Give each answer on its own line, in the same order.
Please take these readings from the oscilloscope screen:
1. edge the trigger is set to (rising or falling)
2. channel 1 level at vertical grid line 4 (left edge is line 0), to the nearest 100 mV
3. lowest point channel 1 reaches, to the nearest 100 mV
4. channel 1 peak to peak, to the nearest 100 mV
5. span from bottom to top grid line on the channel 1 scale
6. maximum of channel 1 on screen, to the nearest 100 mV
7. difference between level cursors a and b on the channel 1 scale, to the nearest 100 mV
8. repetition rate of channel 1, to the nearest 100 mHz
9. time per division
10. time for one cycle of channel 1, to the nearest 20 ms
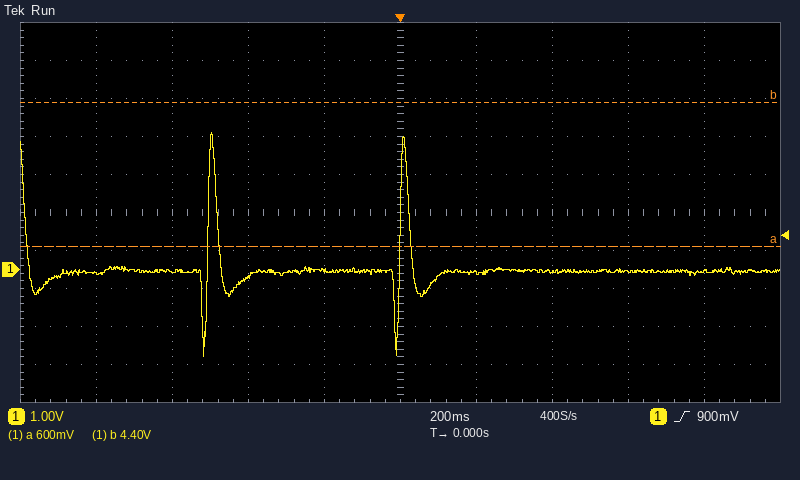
rising
0.0 V
-2.3 V
5.9 V
10 V
3.6 V
3.8 V
2.0 Hz
200 ms
500 ms
